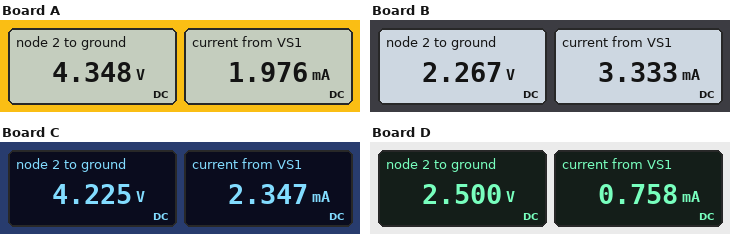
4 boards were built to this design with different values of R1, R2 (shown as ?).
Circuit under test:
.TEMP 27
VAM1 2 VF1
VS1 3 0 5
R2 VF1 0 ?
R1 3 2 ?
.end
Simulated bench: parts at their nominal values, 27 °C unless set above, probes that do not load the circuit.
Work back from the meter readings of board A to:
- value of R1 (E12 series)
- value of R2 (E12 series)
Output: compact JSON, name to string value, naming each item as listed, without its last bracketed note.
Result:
{"value of R1": "330 Ω", "value of R2": "2.2 kΩ"}
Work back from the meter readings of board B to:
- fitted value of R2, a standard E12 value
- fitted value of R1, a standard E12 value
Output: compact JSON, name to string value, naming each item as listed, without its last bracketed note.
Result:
{"fitted value of R2, a standard E12 value": "680 Ω", "fitted value of R1, a standard E12 value": "820 Ω"}
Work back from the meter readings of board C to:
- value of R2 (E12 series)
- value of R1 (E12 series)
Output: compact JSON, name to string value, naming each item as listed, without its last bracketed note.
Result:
{"value of R2": "1.8 kΩ", "value of R1": "330 Ω"}
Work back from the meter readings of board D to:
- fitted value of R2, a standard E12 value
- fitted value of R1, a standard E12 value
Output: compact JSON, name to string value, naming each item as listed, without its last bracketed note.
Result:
{"fitted value of R2, a standard E12 value": "3.3 kΩ", "fitted value of R1, a standard E12 value": "3.3 kΩ"}
